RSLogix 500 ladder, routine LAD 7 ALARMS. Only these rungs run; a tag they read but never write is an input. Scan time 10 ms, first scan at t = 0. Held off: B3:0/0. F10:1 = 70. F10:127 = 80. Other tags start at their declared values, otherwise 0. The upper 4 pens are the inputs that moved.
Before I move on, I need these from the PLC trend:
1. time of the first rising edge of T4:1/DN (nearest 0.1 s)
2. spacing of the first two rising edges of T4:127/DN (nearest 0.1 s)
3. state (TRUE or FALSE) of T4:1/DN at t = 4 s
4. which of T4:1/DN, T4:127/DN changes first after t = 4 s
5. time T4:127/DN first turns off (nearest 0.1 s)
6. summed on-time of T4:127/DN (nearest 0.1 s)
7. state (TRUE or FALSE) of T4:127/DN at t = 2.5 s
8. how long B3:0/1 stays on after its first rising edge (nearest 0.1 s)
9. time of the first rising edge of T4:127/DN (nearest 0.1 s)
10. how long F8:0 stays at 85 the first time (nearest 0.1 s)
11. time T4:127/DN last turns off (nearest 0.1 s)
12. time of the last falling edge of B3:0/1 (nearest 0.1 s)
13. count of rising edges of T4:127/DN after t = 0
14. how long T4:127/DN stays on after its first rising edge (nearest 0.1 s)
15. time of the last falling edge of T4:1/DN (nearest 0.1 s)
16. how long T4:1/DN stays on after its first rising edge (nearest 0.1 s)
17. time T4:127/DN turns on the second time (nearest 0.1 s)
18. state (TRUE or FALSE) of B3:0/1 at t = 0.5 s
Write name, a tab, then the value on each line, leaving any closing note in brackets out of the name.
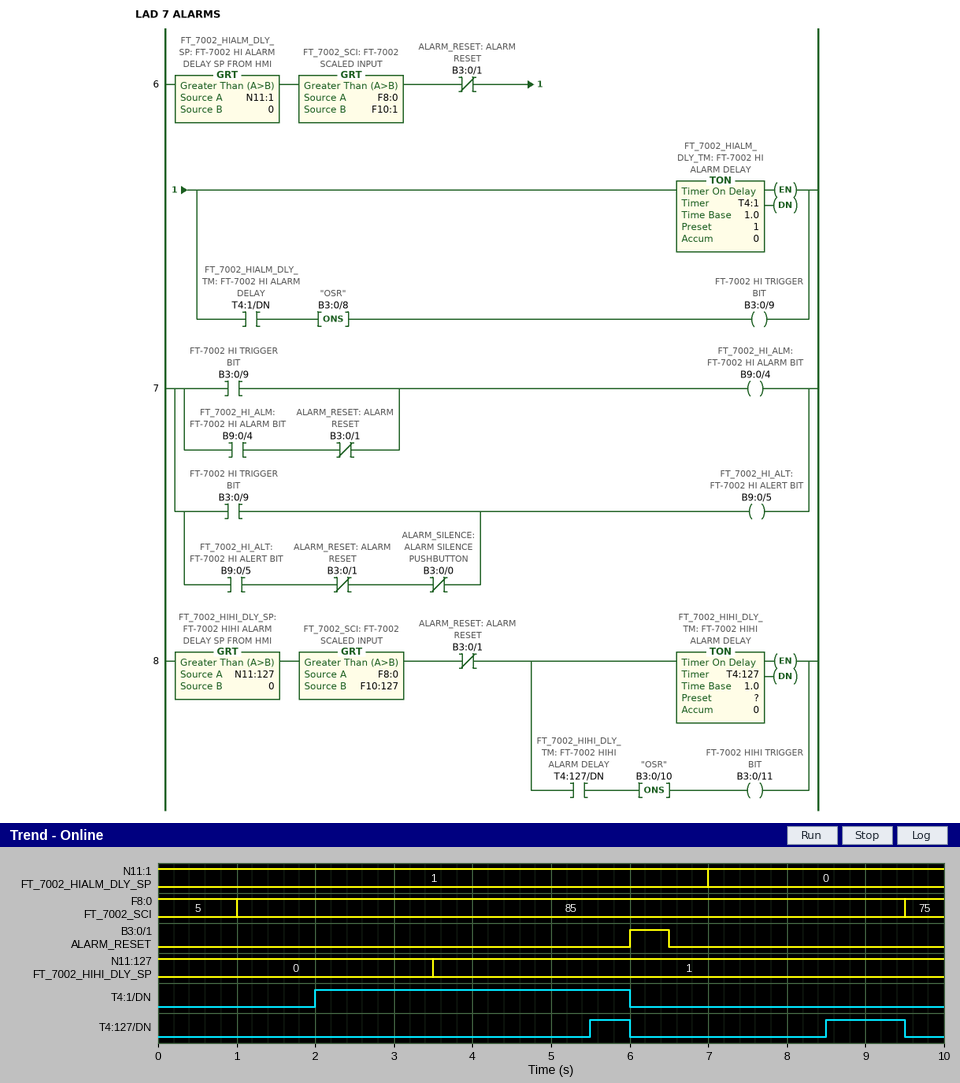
time of the first rising edge of T4:1/DN	2.0 s
spacing of the first two rising edges of T4:127/DN	3.0 s
state (TRUE or FALSE) of T4:1/DN at t = 4 s	TRUE
which of T4:1/DN, T4:127/DN changes first after t = 4 s	T4:127/DN
time T4:127/DN first turns off	6.0 s
summed on-time of T4:127/DN	1.5 s
state (TRUE or FALSE) of T4:127/DN at t = 2.5 s	FALSE
how long B3:0/1 stays on after its first rising edge	0.5 s
time of the first rising edge of T4:127/DN	5.5 s
how long F8:0 stays at 85 the first time	8.5 s
time T4:127/DN last turns off	9.5 s
time of the last falling edge of B3:0/1	6.5 s
count of rising edges of T4:127/DN after t = 0	2
how long T4:127/DN stays on after its first rising edge	0.5 s
time of the last falling edge of T4:1/DN	6.0 s
how long T4:1/DN stays on after its first rising edge	4.0 s
time T4:127/DN turns on the second time	8.5 s
state (TRUE or FALSE) of B3:0/1 at t = 0.5 s	FALSE
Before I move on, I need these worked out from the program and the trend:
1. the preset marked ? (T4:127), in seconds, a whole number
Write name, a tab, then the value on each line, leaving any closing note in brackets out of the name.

the preset marked ? (T4:127), in seconds, a whole number	2 s
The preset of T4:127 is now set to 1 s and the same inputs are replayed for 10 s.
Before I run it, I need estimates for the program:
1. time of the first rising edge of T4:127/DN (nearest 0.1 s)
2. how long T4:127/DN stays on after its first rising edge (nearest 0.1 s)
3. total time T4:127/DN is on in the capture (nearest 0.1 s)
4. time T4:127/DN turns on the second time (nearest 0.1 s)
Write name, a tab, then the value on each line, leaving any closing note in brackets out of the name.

time of the first rising edge of T4:127/DN	4.5 s
how long T4:127/DN stays on after its first rising edge	1.5 s
total time T4:127/DN is on in the capture	3.5 s
time T4:127/DN turns on the second time	7.5 s
